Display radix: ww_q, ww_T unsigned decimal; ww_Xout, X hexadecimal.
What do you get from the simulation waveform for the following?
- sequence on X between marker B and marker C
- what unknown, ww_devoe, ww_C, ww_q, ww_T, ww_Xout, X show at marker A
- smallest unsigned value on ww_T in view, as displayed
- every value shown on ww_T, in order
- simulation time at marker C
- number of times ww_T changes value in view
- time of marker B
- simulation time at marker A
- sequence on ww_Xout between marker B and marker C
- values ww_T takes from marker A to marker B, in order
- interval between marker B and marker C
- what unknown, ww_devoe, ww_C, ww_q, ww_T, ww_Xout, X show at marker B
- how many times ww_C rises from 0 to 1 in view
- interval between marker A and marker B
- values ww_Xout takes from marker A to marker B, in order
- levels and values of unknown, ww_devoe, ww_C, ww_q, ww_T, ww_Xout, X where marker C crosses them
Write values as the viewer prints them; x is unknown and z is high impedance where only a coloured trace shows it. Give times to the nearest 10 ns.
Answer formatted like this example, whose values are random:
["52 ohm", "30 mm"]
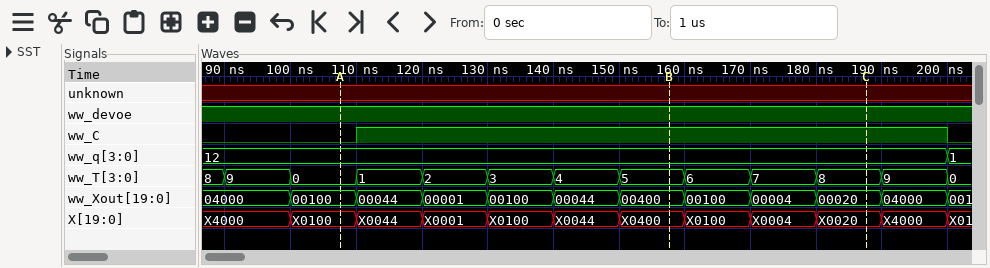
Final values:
["X0400, X0100, X0004, X0020", "unknown=x, ww_devoe=1, ww_C=0, ww_q=12, ww_T=0, ww_Xout=00100, X=X0100", "0", "8, 9, 0, 1, 2, 3, 4, 5, 6, 7, 8, 9, 0", "190 ns", "12", "160 ns", "110 ns", "00400, 00100, 00004, 00020", "0, 1, 2, 3, 4, 5", "30 ns", "unknown=x, ww_devoe=1, ww_C=1, ww_q=12, ww_T=5, ww_Xout=00400, X=X0400", "1", "50 ns", "00100, 00044, 00001, 00100, 00044, 00400", "unknown=x, ww_devoe=1, ww_C=1, ww_q=12, ww_T=8, ww_Xout=00020, X=X0020"]
